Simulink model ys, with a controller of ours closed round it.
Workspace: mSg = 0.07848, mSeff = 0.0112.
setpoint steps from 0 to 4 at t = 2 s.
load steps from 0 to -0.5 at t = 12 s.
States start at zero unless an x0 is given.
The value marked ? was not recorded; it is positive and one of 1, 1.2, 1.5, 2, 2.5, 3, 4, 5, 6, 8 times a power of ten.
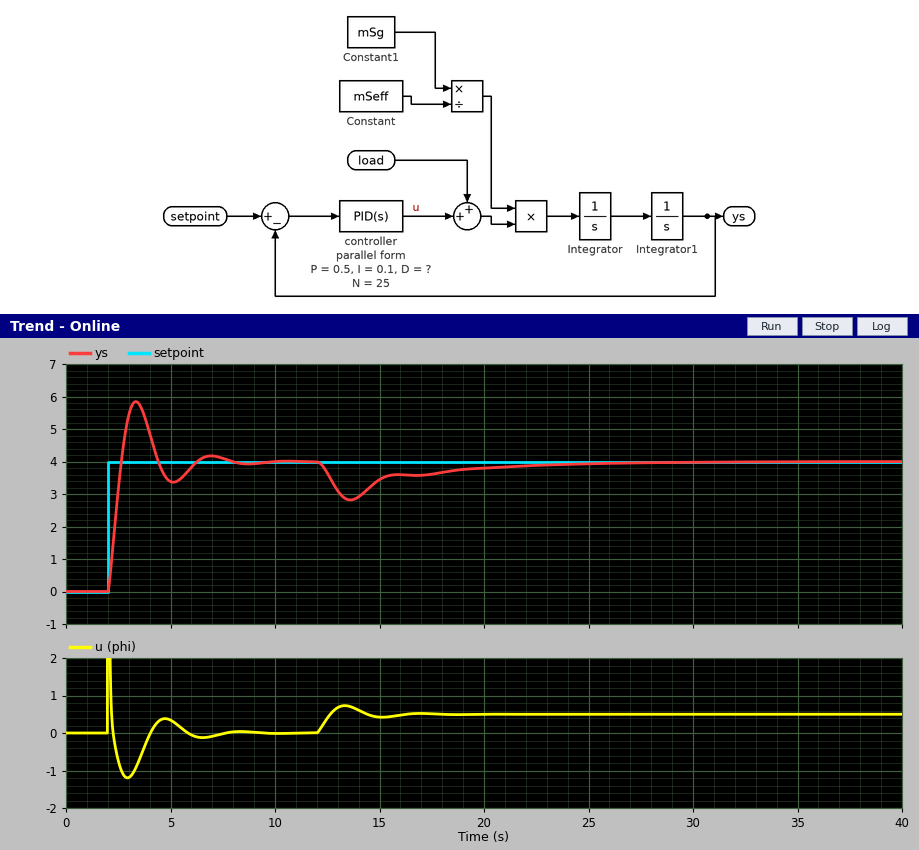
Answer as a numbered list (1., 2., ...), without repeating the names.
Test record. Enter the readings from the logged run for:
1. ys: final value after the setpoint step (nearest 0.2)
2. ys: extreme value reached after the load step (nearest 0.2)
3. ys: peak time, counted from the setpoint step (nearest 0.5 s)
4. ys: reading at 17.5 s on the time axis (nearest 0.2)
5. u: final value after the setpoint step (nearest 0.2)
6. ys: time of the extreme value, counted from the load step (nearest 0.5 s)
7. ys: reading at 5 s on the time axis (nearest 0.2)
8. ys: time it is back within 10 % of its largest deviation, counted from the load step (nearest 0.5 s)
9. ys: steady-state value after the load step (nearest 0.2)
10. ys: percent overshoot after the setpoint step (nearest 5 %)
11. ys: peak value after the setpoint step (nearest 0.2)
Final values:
1. 4.0
2. 2.8
3. 1.5 s
4. 3.6
5. 0.0
6. 1.5 s
7. 3.4
8. 10.5 s
9. 4.0
10. 45 %
11. 5.8
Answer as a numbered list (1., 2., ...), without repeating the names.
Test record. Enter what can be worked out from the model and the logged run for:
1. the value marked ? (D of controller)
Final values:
1. 0.2
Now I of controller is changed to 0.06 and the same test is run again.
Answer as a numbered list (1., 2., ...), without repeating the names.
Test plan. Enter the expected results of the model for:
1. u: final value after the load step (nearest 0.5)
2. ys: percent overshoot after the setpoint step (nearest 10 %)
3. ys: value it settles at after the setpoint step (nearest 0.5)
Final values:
1. 0.5
2. 40 %
3. 4.0
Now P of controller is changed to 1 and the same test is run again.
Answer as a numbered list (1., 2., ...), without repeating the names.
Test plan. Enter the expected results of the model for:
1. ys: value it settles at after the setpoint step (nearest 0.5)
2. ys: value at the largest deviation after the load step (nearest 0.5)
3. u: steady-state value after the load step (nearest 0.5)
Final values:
1. 4.0
2. 3.5
3. 0.5
